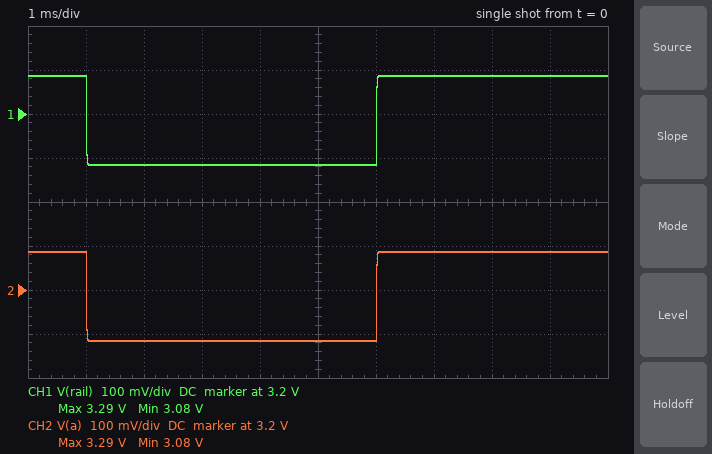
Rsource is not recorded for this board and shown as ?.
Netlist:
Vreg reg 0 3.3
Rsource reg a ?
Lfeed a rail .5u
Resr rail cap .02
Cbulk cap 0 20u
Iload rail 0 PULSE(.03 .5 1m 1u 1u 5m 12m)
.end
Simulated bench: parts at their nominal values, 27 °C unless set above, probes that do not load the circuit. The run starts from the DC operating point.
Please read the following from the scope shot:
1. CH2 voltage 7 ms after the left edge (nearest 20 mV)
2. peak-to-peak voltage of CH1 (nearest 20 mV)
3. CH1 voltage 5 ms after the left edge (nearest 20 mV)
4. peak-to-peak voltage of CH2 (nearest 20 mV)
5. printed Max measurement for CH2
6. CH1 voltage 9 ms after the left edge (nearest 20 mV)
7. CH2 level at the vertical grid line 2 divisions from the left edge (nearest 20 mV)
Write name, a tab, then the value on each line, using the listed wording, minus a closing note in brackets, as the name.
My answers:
CH2 voltage 7 ms after the left edge	3.28 V
peak-to-peak voltage of CH1	200 mV
CH1 voltage 5 ms after the left edge	3.08 V
peak-to-peak voltage of CH2	200 mV
printed Max measurement for CH2	3.29 V
CH1 voltage 9 ms after the left edge	3.28 V
CH2 level at the vertical grid line 2 divisions from the left edge	3.08 V
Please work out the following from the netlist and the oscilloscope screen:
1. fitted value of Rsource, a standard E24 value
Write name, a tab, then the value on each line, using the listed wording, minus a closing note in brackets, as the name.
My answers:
fitted value of Rsource, a standard E24 value	0.43 Ω
